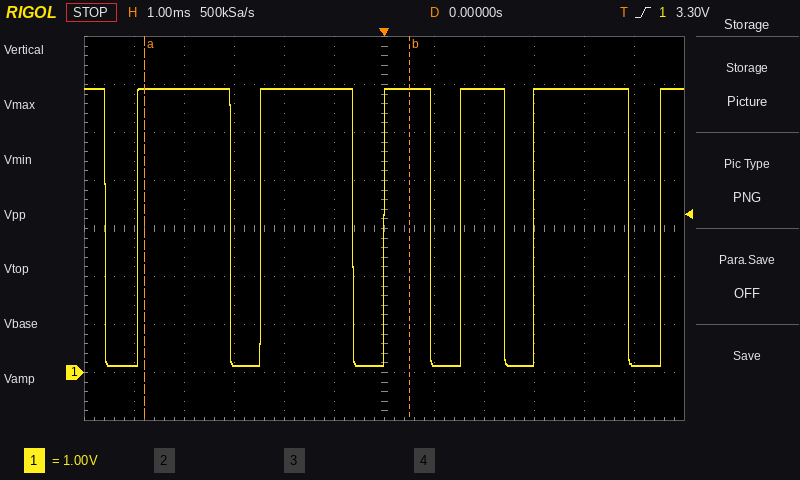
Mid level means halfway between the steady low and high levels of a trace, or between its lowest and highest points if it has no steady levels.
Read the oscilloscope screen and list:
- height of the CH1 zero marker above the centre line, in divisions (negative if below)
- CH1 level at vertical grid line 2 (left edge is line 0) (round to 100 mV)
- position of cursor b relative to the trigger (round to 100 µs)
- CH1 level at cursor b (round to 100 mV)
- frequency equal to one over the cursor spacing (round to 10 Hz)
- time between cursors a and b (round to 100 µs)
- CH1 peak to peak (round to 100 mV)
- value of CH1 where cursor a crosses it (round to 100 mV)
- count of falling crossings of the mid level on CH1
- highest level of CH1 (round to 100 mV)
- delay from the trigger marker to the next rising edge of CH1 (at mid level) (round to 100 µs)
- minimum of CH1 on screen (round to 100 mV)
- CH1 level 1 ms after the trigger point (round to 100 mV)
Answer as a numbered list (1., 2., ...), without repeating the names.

1. -3.0 div
2. 5.9 V
3. +500 µs
4. 5.9 V
5. 190 Hz
6. 5.3 ms
7. 5.8 V
8. 5.9 V
9. 6
10. 5.9 V
11. 1.5 ms
12. 100 mV
13. 200 mV
